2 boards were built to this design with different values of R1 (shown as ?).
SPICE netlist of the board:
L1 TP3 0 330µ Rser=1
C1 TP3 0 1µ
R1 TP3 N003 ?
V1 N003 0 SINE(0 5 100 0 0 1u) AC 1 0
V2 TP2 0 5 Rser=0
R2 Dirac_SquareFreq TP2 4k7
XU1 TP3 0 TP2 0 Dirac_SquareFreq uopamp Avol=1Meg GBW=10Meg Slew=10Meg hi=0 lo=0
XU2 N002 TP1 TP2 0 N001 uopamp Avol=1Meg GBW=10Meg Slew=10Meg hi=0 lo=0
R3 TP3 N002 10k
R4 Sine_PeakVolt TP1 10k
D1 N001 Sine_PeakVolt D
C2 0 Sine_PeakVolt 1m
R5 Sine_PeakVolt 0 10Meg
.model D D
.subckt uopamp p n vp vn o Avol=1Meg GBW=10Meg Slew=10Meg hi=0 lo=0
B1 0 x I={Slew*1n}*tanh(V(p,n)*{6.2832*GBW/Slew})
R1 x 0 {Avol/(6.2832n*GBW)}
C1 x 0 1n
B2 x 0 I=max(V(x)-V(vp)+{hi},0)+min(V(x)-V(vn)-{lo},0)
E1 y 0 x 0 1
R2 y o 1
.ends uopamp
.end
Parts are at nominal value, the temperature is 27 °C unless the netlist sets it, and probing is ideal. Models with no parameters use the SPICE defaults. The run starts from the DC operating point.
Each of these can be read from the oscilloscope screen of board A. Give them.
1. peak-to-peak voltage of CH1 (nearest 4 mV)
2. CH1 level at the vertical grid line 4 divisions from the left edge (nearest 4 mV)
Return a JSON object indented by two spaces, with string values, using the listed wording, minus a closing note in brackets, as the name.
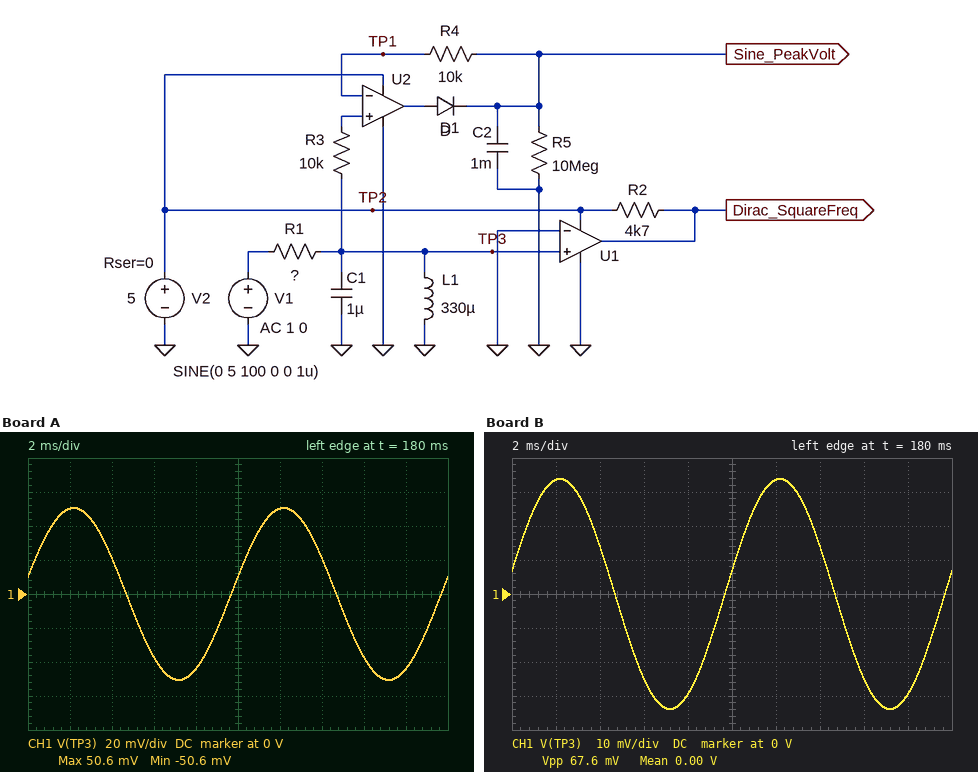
{
  "peak-to-peak voltage of CH1": "100 mV",
  "CH1 level at the vertical grid line 4 divisions from the left edge": "-44 mV"
}
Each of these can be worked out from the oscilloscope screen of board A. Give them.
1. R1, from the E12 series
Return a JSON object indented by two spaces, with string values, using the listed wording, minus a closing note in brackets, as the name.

{
  "R1, from the E12 series": "100 Ω"
}
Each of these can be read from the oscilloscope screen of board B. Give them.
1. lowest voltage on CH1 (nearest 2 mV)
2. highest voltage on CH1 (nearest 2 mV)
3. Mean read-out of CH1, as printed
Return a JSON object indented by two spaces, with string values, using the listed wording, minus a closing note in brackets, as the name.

{
  "lowest voltage on CH1": "-34 mV",
  "highest voltage on CH1": "34 mV",
  "Mean read-out of CH1, as printed": "0.00 V"
}
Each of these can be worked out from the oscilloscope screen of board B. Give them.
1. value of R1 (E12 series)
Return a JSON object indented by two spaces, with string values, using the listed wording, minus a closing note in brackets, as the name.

{
  "value of R1": "150 Ω"
}
